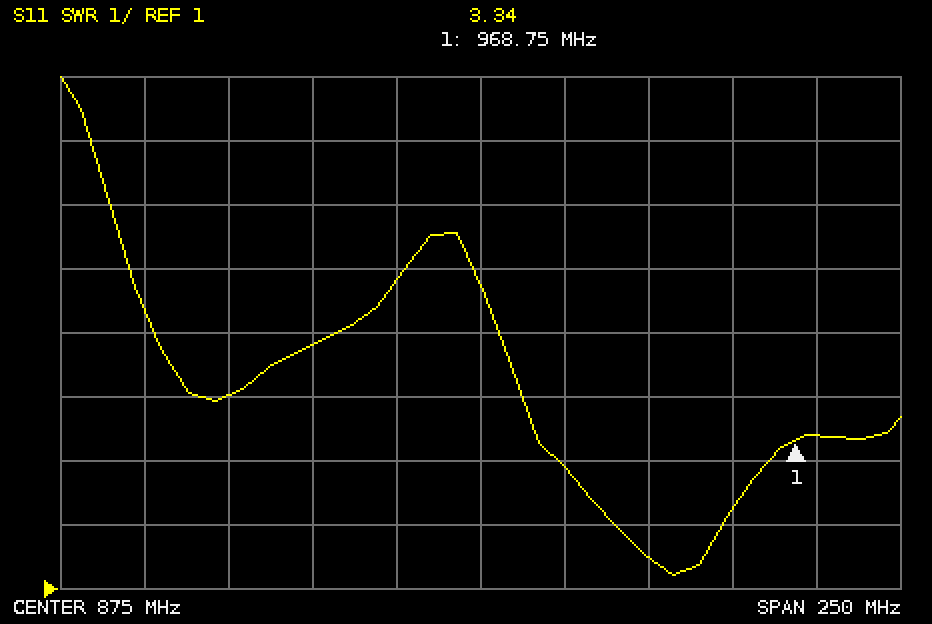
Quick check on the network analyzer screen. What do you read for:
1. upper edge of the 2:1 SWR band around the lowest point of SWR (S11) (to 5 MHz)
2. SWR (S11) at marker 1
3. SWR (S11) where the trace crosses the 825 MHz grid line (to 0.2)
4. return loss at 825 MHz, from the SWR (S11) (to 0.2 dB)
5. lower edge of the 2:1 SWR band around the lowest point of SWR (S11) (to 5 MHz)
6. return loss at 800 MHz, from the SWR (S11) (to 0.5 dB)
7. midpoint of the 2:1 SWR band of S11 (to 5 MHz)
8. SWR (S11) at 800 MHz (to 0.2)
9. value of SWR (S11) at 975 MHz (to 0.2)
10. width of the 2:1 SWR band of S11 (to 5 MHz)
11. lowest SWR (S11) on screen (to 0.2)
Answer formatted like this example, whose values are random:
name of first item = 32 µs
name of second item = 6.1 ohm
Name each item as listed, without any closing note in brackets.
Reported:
upper edge of the 2:1 SWR band around the lowest point of SWR (S11) = 945 MHz
SWR (S11) at marker 1 = 3.34
SWR (S11) where the trace crosses the 825 MHz grid line = 4.8
return loss at 825 MHz, from the SWR (S11) = 3.6 dB
lower edge of the 2:1 SWR band around the lowest point of SWR (S11) = 915 MHz
return loss at 800 MHz, from the SWR (S11) = 4.5 dB
midpoint of the 2:1 SWR band of S11 = 930 MHz
SWR (S11) at 800 MHz = 4.0
value of SWR (S11) at 975 MHz = 3.4
width of the 2:1 SWR band of S11 = 30 MHz
lowest SWR (S11) on screen = 1.2
